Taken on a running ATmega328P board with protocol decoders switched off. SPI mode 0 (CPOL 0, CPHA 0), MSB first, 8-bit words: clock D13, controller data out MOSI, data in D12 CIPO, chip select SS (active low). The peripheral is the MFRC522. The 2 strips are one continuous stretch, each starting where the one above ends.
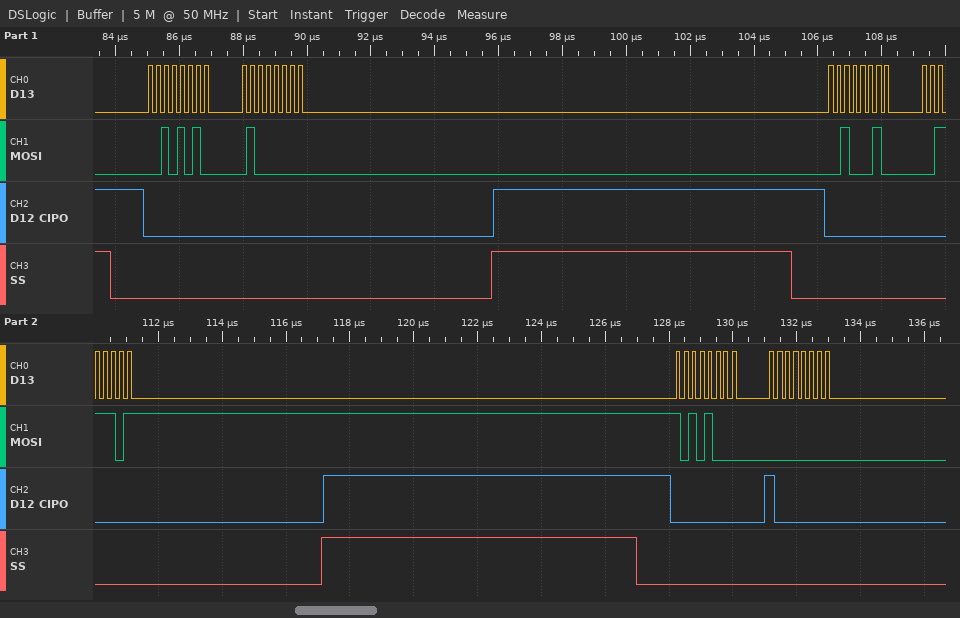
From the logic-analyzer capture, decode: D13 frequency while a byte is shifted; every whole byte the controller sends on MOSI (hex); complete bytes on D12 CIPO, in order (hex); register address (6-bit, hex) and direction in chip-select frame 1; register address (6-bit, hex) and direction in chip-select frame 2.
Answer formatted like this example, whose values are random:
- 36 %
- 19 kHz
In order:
- 4 MHz
- 0x2A 0x40 0x22 0x3D 0xA8 0x00
- 0x00 0x00 0x00 0x00 0x00 0x80
- 0x15 write
- 0x11 write
